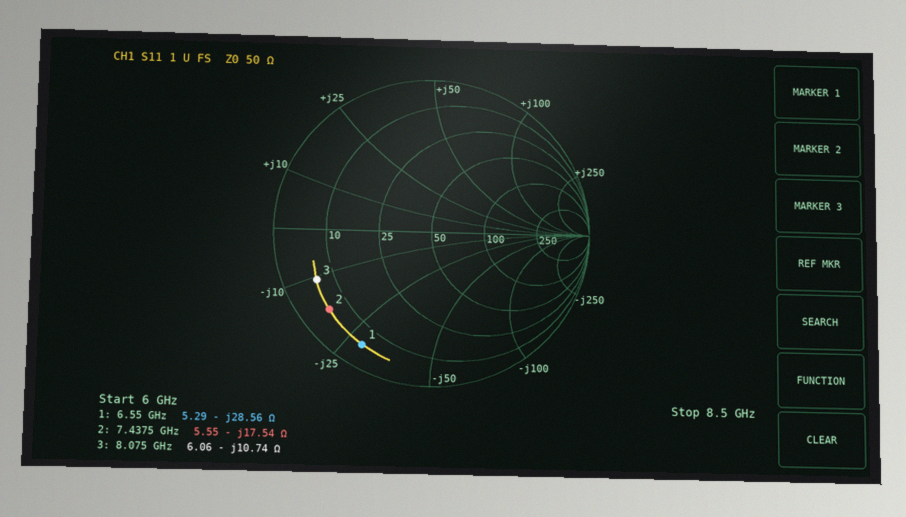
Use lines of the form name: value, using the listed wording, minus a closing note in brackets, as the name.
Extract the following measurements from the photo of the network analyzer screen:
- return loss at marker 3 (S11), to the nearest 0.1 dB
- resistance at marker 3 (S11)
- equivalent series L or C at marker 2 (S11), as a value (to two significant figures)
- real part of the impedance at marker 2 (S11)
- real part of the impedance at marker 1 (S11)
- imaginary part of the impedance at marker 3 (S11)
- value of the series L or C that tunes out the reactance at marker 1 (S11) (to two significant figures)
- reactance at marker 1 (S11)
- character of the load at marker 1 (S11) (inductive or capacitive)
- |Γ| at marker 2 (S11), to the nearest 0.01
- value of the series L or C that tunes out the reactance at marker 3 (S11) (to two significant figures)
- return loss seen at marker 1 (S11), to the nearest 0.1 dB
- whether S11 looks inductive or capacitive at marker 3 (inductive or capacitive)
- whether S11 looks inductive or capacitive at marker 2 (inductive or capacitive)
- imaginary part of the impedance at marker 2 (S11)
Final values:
return loss at marker 3 (S11), to the nearest 0.1 dB: 2.0 dB
resistance at marker 3: 6.06 Ω
equivalent series L or C at marker 2 (S11), as a value: 1.2 pF
real part of the impedance at marker 2: 5.55 Ω
real part of the impedance at marker 1: 5.29 Ω
imaginary part of the impedance at marker 3: -10.74 Ω
value of the series L or C that tunes out the reactance at marker 1 (S11): 690 pH
reactance at marker 1: -28.56 Ω
character of the load at marker 1 (S11): capacitive
|Γ| at marker 2 (S11), to the nearest 0.01: 0.82
value of the series L or C that tunes out the reactance at marker 3 (S11): 210 pH
return loss seen at marker 1 (S11), to the nearest 0.1 dB: 1.4 dB
whether S11 looks inductive or capacitive at marker 3: capacitive
whether S11 looks inductive or capacitive at marker 2: capacitive
imaginary part of the impedance at marker 2: -17.54 Ω
